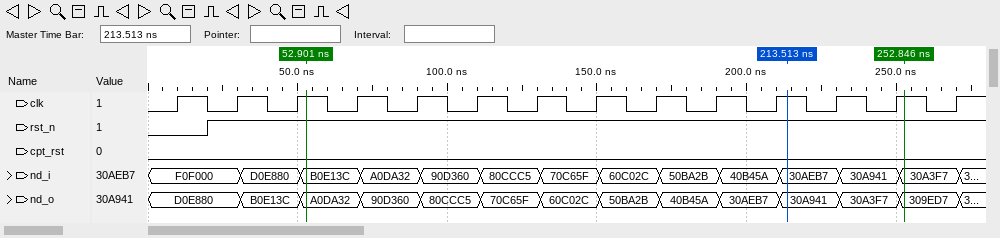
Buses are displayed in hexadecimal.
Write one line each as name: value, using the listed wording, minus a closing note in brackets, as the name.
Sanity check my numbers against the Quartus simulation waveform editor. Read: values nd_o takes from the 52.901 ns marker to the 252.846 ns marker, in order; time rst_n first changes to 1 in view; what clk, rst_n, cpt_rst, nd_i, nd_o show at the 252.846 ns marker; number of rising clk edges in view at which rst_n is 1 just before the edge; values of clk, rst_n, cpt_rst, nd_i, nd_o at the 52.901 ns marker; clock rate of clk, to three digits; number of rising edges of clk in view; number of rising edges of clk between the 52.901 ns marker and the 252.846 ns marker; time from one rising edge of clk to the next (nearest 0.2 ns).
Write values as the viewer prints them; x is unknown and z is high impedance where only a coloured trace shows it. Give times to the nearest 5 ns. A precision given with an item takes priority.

values nd_o takes from the 52.901 ns marker to the 252.846 ns marker, in order: A0DA32, 90D360, 80CCC5, 70C65F, 60C02C, 50BA2B, 40B45A, 30AEB7, 30A941, 30A3F7, 309ED7
time rst_n first changes to 1 in view: 20 ns
what clk, rst_n, cpt_rst, nd_i, nd_o show at the 252.846 ns marker: clk=1, rst_n=1, cpt_rst=0, nd_i=30A3F7, nd_o=309ED7
number of rising clk edges in view at which rst_n is 1 just before the edge: 13
values of clk, rst_n, cpt_rst, nd_i, nd_o at the 52.901 ns marker: clk=1, rst_n=1, cpt_rst=0, nd_i=B0E13C, nd_o=A0DA32
clock rate of clk, to three digits: 50.0 MHz
number of rising edges of clk in view: 14
number of rising edges of clk between the 52.901 ns marker and the 252.846 ns marker: 10
time from one rising edge of clk to the next: 20 ns
